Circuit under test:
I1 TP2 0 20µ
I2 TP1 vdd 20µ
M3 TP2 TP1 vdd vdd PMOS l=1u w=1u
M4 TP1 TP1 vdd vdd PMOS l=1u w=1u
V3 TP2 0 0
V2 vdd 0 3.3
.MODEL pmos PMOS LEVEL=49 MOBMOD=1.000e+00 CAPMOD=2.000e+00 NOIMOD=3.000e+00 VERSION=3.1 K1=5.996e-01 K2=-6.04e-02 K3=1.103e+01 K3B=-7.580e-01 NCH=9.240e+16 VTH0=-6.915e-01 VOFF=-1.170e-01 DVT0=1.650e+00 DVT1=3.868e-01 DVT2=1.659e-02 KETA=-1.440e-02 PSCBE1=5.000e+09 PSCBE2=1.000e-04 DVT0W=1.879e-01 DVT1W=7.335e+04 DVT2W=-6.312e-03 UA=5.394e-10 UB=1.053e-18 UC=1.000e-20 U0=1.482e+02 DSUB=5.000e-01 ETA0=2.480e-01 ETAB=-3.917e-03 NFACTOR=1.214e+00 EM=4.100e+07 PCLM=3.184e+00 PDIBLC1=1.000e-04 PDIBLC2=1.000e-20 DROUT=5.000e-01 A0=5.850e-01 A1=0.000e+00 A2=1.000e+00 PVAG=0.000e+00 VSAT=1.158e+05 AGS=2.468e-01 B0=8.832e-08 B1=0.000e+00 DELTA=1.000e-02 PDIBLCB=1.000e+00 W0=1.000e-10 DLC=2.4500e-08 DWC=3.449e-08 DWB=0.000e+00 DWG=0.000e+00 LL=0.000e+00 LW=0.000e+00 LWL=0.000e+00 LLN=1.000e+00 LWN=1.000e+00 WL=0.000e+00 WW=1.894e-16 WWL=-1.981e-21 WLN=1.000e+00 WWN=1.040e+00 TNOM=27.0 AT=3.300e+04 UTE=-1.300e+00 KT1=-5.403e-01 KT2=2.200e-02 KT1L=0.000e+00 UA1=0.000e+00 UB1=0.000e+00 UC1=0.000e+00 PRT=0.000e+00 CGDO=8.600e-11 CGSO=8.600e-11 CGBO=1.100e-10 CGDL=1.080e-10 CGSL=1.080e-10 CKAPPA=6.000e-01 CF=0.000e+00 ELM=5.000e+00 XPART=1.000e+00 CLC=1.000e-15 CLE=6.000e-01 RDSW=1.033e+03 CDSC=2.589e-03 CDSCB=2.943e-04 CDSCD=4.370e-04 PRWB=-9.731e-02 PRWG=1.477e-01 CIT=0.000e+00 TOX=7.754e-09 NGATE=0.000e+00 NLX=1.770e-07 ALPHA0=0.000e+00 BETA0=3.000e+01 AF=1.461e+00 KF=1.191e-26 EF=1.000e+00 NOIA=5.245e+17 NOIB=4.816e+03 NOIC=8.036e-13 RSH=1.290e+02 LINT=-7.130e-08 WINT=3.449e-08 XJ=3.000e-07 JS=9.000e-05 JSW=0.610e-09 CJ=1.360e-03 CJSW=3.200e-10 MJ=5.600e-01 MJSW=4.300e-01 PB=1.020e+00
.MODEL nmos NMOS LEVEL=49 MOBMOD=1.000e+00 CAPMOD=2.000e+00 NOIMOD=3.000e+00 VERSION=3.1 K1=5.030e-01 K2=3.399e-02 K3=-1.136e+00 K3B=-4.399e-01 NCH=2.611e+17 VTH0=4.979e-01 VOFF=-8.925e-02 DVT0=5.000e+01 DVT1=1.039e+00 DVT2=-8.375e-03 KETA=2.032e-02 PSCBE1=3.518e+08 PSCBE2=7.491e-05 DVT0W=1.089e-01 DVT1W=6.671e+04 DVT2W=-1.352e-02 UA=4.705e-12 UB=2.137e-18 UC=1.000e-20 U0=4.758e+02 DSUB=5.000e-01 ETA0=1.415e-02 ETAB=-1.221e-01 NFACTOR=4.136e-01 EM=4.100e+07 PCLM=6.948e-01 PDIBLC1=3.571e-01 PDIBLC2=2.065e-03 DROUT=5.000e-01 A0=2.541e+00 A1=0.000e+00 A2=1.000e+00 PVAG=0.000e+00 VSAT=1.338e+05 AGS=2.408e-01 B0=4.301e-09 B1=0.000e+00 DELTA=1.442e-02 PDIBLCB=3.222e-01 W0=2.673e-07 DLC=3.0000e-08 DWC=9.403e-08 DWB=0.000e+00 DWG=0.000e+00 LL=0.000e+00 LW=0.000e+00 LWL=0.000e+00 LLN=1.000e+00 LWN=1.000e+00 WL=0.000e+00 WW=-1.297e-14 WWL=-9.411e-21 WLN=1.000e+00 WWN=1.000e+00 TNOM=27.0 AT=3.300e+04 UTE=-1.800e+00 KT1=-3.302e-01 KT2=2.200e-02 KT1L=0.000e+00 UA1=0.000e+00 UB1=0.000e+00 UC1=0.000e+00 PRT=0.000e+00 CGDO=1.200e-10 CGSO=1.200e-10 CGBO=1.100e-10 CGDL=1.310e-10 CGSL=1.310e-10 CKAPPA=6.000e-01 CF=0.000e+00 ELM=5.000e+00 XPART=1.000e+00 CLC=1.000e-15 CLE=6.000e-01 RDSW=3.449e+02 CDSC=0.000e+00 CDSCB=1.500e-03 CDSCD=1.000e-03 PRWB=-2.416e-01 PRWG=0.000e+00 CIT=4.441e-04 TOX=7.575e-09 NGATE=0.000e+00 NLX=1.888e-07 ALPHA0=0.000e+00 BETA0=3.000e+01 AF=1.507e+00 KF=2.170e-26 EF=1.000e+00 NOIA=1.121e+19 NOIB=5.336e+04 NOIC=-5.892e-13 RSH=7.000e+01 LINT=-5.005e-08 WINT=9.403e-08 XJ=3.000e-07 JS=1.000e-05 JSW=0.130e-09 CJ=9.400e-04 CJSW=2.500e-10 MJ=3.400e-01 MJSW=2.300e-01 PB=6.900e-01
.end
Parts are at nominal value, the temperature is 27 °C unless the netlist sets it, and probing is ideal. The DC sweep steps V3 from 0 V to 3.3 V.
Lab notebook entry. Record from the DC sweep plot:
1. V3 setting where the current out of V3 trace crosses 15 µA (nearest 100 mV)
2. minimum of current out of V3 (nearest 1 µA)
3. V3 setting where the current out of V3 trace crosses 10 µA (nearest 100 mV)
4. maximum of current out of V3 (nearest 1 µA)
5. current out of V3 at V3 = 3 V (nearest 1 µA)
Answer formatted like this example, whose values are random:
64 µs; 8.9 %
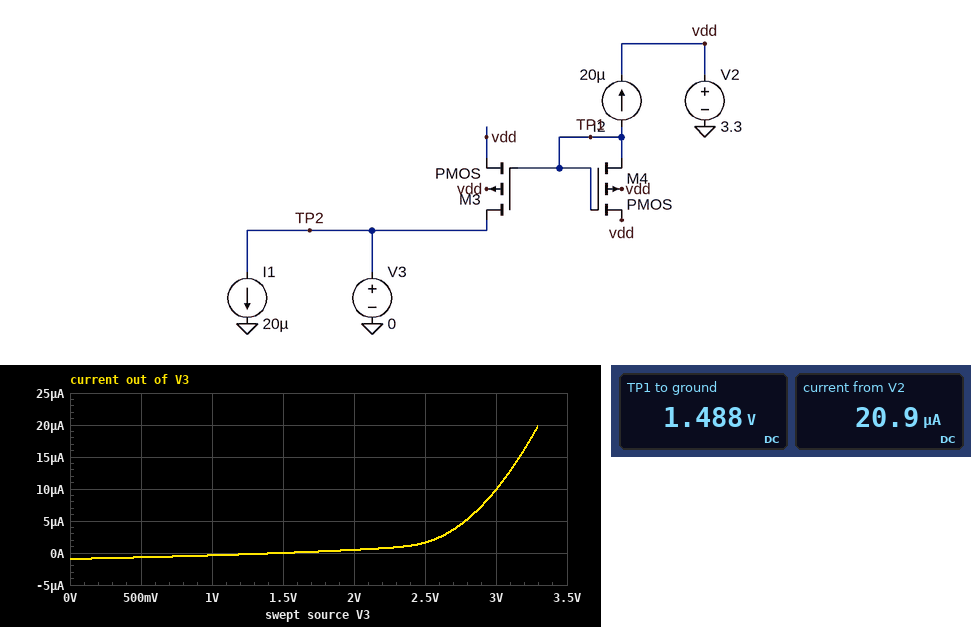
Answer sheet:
3.2 V; -1 µA; 3.0 V; 20 µA; 10 µA
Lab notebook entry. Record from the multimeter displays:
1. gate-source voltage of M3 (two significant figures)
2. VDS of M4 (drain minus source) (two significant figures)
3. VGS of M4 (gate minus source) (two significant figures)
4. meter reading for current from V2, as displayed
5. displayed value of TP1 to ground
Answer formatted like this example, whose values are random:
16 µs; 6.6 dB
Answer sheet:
-1.8 V; -1.8 V; -1.8 V; 20.9 µA; 1.488 V
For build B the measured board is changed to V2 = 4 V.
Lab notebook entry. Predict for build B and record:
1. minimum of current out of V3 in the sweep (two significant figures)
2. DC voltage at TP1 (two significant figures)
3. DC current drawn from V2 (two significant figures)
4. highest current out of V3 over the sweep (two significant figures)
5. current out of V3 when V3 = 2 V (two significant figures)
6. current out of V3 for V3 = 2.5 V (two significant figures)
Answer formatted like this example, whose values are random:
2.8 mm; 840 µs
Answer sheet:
-1.2 µA; 2.2 V; 21 µA; 2.4 µA; -150 nA; 280 nA
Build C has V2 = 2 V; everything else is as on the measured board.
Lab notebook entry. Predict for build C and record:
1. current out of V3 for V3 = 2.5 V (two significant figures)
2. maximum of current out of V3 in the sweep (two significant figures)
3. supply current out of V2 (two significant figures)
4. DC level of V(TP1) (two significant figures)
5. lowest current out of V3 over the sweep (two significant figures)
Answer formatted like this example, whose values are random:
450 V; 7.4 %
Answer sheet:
47 µA; 170 µA; 20 µA; 190 mV; -150 nA
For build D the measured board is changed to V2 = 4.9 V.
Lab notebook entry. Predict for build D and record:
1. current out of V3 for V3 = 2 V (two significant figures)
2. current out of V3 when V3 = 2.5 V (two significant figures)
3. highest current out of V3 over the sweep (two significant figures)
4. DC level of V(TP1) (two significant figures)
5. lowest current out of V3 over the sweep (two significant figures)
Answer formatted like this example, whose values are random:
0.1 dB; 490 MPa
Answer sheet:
-730 nA; -430 nA; 190 nA; 3.1 V; -1.5 µA
